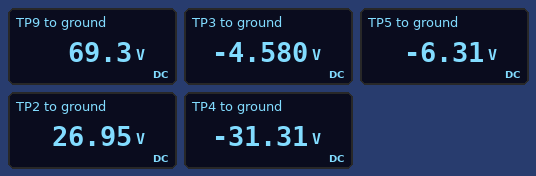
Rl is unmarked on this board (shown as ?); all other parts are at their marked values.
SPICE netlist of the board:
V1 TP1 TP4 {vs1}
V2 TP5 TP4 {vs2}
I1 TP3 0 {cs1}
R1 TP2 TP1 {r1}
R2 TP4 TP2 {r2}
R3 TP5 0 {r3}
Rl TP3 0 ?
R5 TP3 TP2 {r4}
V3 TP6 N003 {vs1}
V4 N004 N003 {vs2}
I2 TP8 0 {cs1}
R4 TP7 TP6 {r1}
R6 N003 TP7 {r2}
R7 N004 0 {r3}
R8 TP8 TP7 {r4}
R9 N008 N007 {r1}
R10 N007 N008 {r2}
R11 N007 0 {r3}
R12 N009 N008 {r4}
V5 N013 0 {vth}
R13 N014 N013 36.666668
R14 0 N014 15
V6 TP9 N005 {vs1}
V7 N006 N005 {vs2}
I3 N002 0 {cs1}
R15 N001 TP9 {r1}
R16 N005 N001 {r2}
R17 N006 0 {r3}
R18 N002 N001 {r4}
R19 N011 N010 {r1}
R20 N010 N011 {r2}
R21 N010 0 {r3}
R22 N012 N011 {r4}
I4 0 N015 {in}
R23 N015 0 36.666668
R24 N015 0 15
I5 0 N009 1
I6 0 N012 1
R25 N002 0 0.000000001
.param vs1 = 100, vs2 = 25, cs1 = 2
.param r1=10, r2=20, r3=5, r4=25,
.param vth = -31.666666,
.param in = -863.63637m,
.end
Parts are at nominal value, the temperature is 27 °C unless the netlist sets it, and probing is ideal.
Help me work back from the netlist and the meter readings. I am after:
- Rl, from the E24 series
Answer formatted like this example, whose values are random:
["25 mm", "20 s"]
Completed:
["6.2 Ω"]
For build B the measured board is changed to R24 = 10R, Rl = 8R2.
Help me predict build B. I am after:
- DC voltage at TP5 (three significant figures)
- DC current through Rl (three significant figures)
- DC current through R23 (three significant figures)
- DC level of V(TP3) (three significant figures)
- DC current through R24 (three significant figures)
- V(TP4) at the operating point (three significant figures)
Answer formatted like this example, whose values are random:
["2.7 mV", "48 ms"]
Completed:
["-6.47 V", "706 mA", "185 mA", "-5.79 V", "679 mA", "-31.5 V"]
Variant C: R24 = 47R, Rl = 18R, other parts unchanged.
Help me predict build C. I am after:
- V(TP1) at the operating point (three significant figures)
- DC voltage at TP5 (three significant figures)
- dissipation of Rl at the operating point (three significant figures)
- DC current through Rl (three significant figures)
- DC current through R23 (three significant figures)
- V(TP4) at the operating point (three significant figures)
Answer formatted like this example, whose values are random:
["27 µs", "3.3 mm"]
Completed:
["67.9 V", "-7.10 V", "6.04 W", "579 mA", "485 mA", "-32.1 V"]
